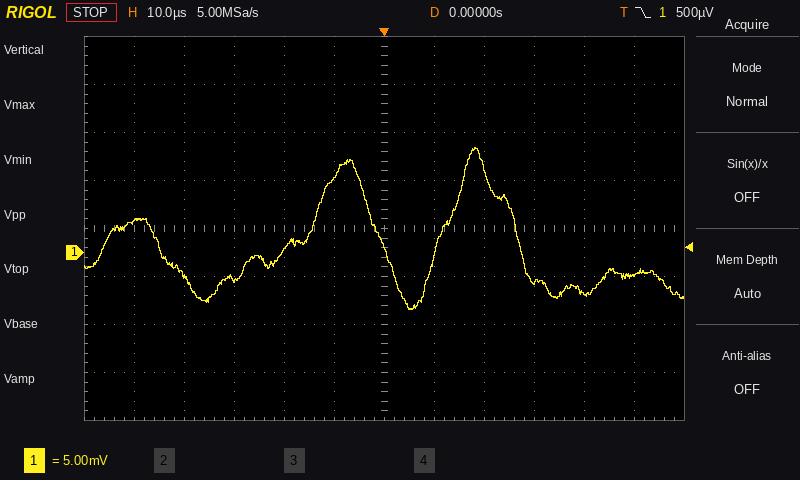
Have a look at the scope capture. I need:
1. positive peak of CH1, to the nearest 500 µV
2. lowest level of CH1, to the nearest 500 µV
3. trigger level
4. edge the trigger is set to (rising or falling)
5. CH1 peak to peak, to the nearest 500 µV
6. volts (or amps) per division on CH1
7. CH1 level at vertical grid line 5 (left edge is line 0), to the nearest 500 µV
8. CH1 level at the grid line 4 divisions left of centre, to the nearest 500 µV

11.0 mV
-6.0 mV
500 µV
falling
17.0 mV
5 mV
8.0 mV
-2.5 mV
